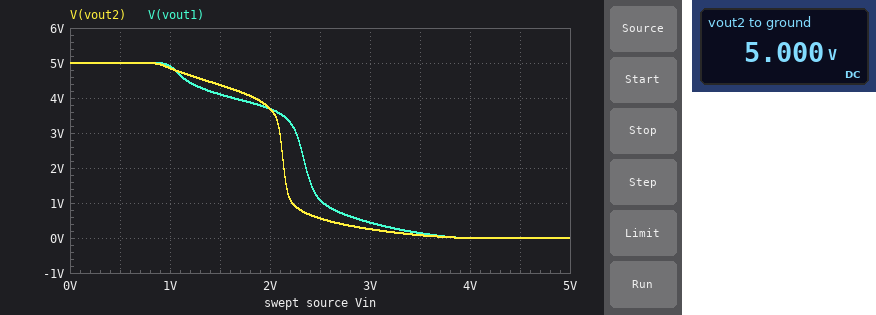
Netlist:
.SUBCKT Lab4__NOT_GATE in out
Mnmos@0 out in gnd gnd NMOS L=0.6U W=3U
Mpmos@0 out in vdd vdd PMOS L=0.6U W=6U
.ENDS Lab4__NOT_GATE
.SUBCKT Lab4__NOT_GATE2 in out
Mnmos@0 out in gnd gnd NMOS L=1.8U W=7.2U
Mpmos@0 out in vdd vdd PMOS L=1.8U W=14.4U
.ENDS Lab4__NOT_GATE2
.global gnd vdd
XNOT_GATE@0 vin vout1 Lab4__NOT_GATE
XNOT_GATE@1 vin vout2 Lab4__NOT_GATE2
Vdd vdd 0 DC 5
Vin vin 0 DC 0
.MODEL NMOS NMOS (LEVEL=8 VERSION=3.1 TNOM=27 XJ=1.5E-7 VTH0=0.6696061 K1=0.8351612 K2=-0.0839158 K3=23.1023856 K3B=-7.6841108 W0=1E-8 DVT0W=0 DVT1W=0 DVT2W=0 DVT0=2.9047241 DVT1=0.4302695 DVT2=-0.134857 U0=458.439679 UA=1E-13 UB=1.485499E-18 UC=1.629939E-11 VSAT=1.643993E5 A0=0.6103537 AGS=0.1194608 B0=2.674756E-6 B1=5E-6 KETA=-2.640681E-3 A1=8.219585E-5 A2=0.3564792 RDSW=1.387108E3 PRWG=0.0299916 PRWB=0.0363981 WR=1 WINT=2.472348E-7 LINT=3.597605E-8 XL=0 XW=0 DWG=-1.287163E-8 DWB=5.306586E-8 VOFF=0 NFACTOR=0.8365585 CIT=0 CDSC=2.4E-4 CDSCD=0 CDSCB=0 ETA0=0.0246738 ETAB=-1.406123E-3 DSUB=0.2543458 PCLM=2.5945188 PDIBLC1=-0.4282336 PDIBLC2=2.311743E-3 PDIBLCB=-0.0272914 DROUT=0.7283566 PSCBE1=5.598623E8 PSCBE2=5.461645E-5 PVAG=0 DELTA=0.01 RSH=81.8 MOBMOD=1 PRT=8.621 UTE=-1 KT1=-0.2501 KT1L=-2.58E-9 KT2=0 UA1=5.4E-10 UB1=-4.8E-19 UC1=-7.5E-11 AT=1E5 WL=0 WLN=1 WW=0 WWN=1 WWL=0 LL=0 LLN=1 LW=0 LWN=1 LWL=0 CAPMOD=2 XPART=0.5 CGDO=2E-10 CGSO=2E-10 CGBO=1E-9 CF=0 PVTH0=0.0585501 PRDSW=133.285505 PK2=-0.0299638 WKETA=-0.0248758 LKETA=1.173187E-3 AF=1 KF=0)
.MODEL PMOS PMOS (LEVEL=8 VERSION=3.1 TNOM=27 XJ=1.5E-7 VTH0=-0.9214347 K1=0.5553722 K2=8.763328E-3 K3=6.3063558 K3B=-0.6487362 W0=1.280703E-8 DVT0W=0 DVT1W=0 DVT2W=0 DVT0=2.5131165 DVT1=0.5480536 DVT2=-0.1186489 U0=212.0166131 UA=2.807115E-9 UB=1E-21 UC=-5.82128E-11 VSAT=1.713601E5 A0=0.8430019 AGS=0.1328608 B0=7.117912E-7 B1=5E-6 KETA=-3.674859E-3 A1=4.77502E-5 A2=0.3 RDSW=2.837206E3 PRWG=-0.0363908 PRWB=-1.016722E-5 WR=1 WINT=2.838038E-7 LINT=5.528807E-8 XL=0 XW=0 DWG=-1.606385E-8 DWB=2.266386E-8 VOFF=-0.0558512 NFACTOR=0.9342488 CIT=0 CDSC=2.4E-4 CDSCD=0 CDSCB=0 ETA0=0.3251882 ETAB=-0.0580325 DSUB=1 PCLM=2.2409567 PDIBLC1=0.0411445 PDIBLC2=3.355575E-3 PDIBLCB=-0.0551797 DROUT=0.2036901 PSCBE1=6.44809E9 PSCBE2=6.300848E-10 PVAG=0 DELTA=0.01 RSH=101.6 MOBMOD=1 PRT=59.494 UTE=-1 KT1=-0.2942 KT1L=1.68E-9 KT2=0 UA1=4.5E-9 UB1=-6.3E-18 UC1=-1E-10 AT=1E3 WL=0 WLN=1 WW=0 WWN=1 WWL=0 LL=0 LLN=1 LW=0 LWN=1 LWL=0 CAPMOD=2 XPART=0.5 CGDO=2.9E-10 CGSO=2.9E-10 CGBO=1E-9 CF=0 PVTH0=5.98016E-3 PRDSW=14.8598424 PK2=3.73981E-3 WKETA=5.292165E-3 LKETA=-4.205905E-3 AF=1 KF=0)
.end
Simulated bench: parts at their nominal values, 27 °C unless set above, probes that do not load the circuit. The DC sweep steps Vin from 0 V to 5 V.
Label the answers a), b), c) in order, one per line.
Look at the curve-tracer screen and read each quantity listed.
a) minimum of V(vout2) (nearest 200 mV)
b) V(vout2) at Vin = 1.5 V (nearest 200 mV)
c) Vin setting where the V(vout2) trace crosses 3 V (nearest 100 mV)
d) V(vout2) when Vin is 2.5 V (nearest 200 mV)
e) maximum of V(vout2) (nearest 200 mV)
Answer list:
a) 0 V
b) 4.4 V
c) 2.1 V
d) 600 mV
e) 5.0 V
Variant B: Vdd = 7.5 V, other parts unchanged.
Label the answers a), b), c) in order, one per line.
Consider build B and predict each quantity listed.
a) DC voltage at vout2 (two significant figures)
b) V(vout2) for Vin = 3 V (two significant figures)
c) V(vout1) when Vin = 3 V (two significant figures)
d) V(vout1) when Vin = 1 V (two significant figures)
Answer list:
a) 7.5 V
b) 5.0 V
c) 4.5 V
d) 7.1 V
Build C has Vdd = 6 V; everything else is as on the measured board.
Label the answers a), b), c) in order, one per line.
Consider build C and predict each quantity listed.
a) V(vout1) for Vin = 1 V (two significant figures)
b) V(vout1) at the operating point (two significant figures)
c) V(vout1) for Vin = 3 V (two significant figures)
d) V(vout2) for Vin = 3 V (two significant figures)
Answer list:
a) 5.8 V
b) 6.0 V
c) 1.7 V
d) 860 mV
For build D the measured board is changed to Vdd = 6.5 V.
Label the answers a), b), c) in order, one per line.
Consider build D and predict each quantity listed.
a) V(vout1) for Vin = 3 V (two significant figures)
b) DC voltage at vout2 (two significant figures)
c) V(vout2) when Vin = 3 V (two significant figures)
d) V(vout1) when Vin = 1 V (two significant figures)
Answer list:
a) 3.7 V
b) 6.5 V
c) 1.5 V
d) 6.2 V
